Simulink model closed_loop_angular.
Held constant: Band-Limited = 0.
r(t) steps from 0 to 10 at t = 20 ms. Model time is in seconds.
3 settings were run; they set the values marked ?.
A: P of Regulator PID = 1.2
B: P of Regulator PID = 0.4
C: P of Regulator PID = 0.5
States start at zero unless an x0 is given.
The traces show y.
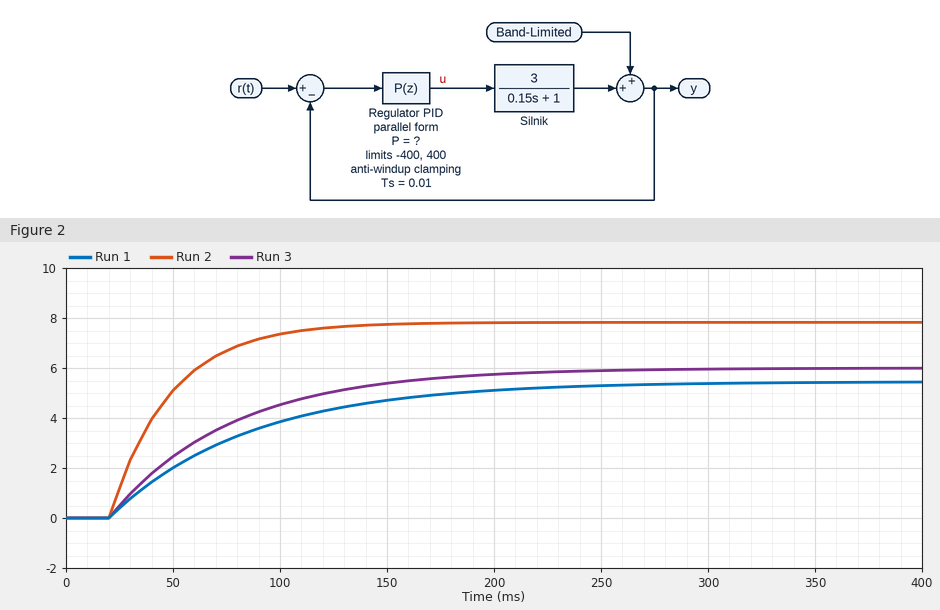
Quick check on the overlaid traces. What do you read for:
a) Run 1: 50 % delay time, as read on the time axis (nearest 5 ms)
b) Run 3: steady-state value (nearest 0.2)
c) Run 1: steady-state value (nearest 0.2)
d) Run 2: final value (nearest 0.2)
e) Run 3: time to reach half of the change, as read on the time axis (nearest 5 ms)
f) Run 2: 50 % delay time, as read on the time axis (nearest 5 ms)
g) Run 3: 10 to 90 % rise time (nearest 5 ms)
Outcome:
65 ms
6.0
5.4
7.8
60 ms
40 ms
125 ms
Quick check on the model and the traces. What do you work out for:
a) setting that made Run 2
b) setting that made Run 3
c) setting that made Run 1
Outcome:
A
C
B
